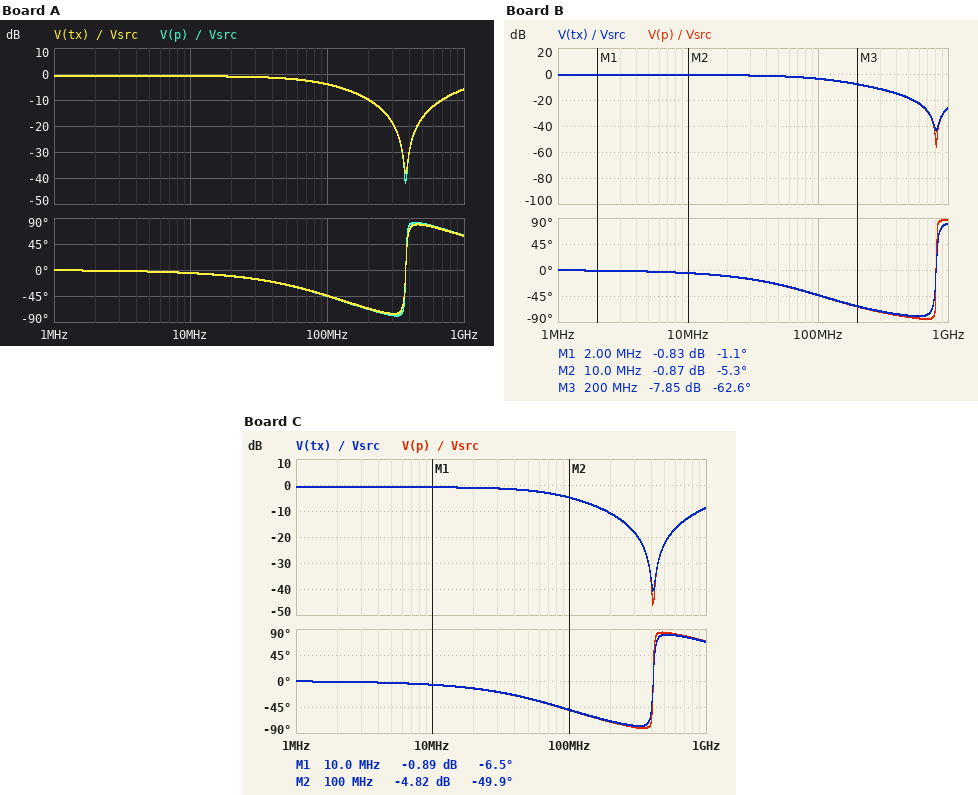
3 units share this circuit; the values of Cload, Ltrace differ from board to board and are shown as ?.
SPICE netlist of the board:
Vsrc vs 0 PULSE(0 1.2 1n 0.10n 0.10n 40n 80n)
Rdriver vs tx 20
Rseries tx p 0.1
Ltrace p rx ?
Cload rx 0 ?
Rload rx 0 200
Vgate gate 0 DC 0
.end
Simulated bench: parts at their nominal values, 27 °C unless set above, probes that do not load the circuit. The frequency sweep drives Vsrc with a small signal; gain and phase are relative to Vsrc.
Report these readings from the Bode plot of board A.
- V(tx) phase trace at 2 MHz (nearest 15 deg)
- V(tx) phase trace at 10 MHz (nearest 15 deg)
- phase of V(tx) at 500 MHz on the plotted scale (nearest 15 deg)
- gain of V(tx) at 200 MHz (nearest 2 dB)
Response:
0 deg
0 deg
75 deg
-10 dB
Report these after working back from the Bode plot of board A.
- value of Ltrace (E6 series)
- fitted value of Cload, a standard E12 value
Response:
2.2 nH
82 pF
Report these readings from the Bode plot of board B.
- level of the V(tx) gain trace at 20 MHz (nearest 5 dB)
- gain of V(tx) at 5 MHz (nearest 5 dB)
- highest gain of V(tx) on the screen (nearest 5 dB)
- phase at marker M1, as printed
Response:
0 dB
0 dB
0 dB
-1.1 deg
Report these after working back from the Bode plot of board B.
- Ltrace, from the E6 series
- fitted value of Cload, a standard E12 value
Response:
470 pH
82 pF
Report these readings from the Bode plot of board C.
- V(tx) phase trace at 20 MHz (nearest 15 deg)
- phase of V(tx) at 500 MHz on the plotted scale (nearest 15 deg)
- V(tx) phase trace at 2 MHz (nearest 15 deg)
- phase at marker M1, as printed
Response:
-15 deg
75 deg
0 deg
-6.5 deg
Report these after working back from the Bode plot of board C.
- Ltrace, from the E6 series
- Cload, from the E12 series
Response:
1.5 nH
100 pF
